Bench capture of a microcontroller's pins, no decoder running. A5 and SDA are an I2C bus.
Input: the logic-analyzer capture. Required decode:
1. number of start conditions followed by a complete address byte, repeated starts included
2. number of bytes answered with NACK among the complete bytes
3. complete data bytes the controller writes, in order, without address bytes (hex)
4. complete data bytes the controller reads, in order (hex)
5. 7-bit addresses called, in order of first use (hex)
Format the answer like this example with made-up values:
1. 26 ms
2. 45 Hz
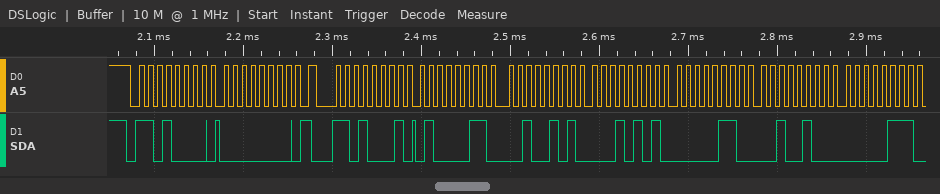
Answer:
1. 2
2. 0
3. 00
4. 43 25 15 06 24 07
5. 0x68
